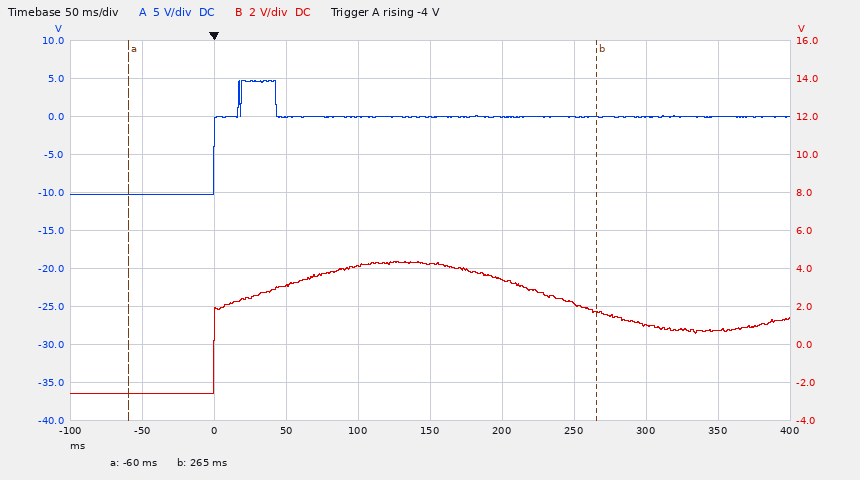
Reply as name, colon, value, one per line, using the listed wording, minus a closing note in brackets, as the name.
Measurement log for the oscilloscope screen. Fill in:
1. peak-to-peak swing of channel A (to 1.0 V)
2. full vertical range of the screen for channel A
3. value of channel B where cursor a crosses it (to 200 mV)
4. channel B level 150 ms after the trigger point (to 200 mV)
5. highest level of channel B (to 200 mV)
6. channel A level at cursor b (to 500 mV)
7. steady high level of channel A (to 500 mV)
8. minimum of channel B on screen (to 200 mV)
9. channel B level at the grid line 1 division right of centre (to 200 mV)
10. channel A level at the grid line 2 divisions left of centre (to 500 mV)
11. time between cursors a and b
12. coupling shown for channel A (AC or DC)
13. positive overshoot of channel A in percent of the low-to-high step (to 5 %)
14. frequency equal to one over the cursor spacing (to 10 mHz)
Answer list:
peak-to-peak swing of channel A: 15.0 V
full vertical range of the screen for channel A: 50 V
value of channel B where cursor a crosses it: -2.6 V
channel B level 150 ms after the trigger point: 4.2 V
highest level of channel B: 4.4 V
channel A level at cursor b: 0.0 V
steady high level of channel A: 0.0 V
minimum of channel B on screen: -2.6 V
channel B level at the grid line 1 division right of centre: 3.4 V
channel A level at the grid line 2 divisions left of centre: 0.0 V
time between cursors a and b: 325 ms
coupling shown for channel A: DC
positive overshoot of channel A in percent of the low-to-high step: 45 %
frequency equal to one over the cursor spacing: 3.08 Hz
